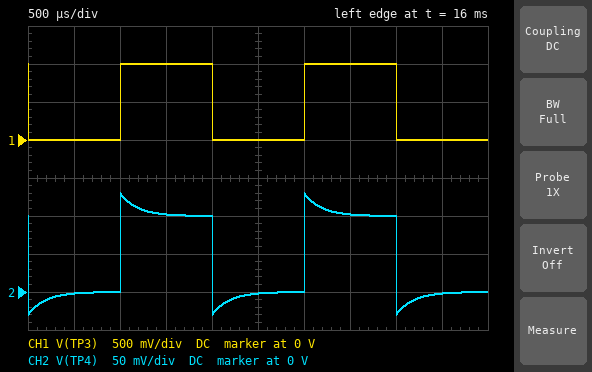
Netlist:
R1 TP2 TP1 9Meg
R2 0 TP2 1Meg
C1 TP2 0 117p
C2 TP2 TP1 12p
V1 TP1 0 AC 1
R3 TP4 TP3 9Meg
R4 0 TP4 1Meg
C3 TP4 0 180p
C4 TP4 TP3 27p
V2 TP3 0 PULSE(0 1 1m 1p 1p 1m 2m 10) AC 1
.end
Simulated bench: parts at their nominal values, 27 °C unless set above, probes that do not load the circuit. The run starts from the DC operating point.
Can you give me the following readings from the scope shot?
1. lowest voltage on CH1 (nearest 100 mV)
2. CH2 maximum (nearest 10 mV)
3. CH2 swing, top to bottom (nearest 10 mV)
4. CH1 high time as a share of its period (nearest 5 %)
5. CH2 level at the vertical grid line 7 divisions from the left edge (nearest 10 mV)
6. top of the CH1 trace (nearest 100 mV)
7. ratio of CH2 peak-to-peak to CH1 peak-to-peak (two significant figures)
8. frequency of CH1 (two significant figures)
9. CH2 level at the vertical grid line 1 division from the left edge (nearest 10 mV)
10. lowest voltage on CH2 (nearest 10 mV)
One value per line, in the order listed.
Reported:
0 V
130 mV
160 mV
50 %
100 mV
1.0 V
0.16
500 Hz
0 V
-30 mV
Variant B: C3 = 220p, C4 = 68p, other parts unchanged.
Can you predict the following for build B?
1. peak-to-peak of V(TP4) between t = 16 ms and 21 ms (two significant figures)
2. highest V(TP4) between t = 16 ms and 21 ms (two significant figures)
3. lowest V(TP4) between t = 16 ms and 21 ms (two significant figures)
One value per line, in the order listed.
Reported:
370 mV
230 mV
-130 mV
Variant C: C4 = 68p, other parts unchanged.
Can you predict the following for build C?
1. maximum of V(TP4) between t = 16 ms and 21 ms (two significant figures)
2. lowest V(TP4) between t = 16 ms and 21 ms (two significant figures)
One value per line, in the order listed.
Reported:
270 mV
-170 mV
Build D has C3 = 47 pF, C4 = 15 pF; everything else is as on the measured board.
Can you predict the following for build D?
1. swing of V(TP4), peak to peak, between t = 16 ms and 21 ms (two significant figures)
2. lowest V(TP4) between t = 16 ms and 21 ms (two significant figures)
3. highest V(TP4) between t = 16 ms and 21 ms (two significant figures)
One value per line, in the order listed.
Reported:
380 mV
-140 mV
240 mV
